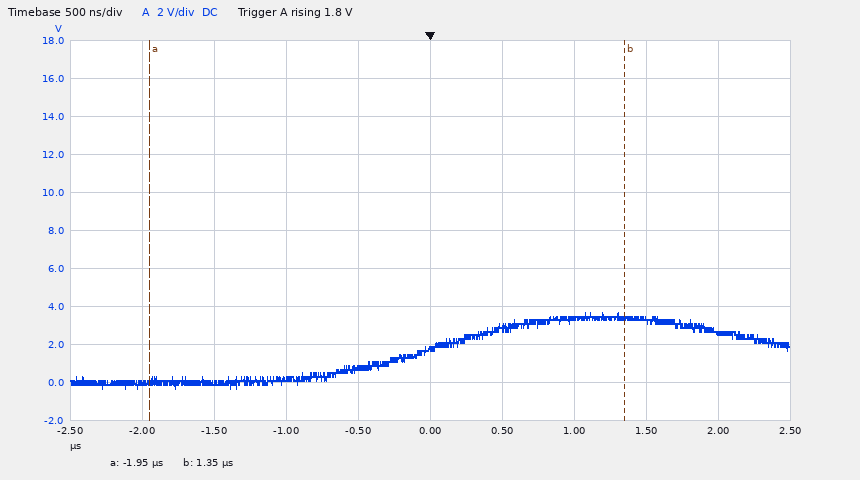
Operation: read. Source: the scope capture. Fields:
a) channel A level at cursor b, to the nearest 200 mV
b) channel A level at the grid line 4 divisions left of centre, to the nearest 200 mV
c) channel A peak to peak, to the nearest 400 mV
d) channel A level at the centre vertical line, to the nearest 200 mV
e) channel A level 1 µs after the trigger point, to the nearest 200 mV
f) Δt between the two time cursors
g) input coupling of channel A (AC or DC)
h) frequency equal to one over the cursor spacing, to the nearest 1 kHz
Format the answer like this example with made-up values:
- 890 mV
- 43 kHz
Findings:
- 3.4 V
- 0.0 V
- 4.0 V
- 1.8 V
- 3.4 V
- 3.30 µs
- DC
- 303 kHz
